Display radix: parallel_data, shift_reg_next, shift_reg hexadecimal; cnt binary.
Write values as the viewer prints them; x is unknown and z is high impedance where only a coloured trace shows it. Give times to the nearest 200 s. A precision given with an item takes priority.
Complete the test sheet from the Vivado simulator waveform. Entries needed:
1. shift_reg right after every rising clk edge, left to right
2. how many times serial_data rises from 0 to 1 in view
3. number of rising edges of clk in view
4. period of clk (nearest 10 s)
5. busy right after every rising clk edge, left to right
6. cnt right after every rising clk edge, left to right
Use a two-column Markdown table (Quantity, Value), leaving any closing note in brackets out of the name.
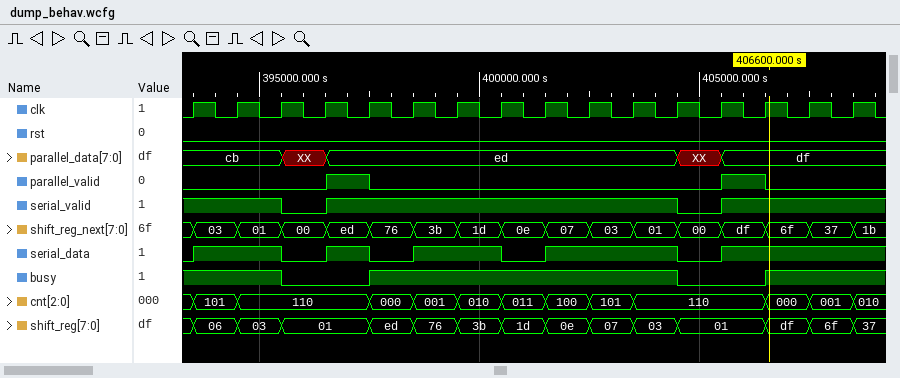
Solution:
| Quantity | Value |
|---|---|
| shift_reg right after every rising clk edge, left to right | 06, 03, 01, 01, ed, 76, 3b, 1d, 0e, 07, 03, 01, 01, df, 6f, 37 |
| how many times serial_data rises from 0 to 1 in view | 5 |
| number of rising edges of clk in view | 16 |
| period of clk | 1000 s |
| busy right after every rising clk edge, left to right | 1 1 0 0 1 1 1 1 1 1 1 0 0 1 1 1 |
| cnt right after every rising clk edge, left to right | 101, 110, 110, 110, 000, 001, 010, 011, 100, 101, 110, 110, 110, 000, 001, 010 |
